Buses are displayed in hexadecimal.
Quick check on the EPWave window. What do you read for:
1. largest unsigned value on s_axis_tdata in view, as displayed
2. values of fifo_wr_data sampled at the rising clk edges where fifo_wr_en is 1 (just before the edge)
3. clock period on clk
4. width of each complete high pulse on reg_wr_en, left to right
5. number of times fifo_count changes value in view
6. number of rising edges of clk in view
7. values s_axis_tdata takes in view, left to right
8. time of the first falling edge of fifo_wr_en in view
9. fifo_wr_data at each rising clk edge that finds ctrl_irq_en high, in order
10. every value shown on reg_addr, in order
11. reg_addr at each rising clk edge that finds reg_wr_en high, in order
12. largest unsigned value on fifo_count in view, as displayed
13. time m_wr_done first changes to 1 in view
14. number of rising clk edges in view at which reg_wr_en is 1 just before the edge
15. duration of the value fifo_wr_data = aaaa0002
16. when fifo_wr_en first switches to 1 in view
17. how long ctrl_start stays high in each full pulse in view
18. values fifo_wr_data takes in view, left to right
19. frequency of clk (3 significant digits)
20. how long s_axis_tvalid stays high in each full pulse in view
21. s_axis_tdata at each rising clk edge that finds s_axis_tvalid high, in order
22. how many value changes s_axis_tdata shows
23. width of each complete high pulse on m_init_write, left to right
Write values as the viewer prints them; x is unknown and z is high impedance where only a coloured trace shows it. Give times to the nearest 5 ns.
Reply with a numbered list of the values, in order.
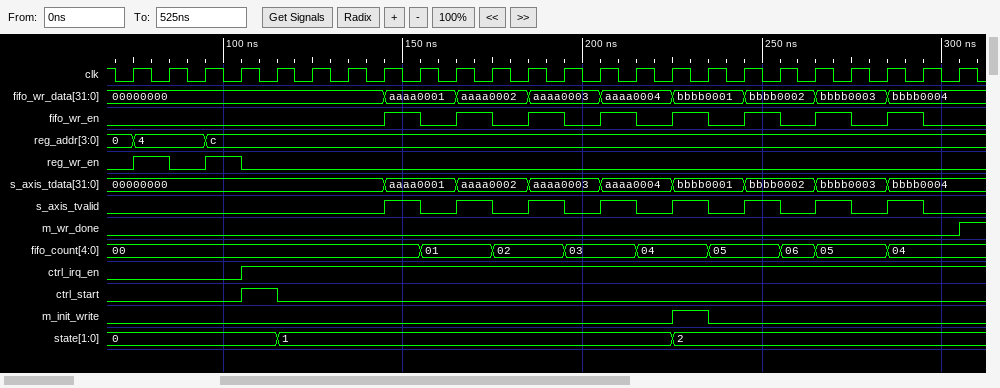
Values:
1. bbbb0004
2. aaaa0001, aaaa0002, aaaa0003, aaaa0004, bbbb0001, bbbb0002, bbbb0003, bbbb0004
3. 10 ns
4. 10 ns, 10 ns
5. 8
6. 24
7. 00000000, aaaa0001, aaaa0002, aaaa0003, aaaa0004, bbbb0001, bbbb0002, bbbb0003, bbbb0004
8. 155 ns
9. 00000000, 00000000, 00000000, 00000000, aaaa0001, aaaa0001, aaaa0002, aaaa0002, aaaa0003, aaaa0003, aaaa0004, aaaa0004, bbbb0001, bbbb0001, bbbb0002, bbbb0002, bbbb0003, bbbb0003, bbbb0004, bbbb0004
10. 0, 4, c
11. 4, c
12. 06
13. 305 ns
14. 2
15. 20 ns
16. 145 ns
17. 10 ns
18. 00000000, aaaa0001, aaaa0002, aaaa0003, aaaa0004, bbbb0001, bbbb0002, bbbb0003, bbbb0004
19. 100 MHz
20. 10 ns, 10 ns, 10 ns, 10 ns, 10 ns, 10 ns, 10 ns, 10 ns
21. aaaa0001, aaaa0002, aaaa0003, aaaa0004, bbbb0001, bbbb0002, bbbb0003, bbbb0004
22. 8
23. 10 ns
